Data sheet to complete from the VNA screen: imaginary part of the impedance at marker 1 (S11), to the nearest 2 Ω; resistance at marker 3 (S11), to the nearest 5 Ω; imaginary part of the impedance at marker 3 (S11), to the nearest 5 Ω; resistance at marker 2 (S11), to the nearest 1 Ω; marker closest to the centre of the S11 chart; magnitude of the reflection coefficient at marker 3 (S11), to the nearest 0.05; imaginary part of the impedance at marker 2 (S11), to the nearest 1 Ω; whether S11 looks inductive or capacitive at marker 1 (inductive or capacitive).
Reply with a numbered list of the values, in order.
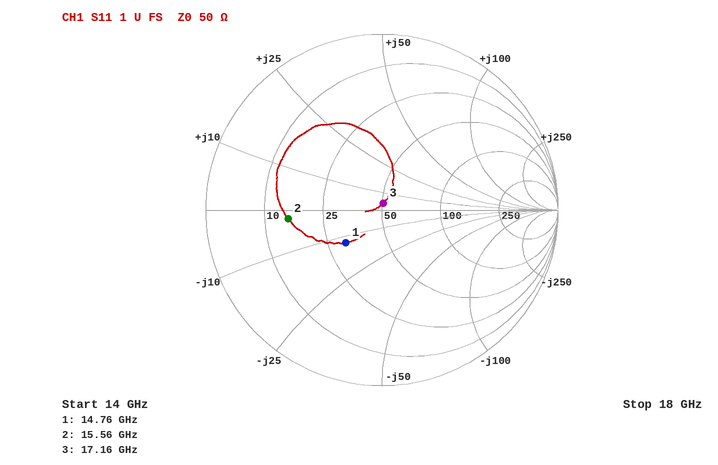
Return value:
1. -12 Ω
2. 50 Ω
3. +5 Ω
4. 15 Ω
5. marker 3
6. 0.05
7. -2 Ω
8. capacitive
